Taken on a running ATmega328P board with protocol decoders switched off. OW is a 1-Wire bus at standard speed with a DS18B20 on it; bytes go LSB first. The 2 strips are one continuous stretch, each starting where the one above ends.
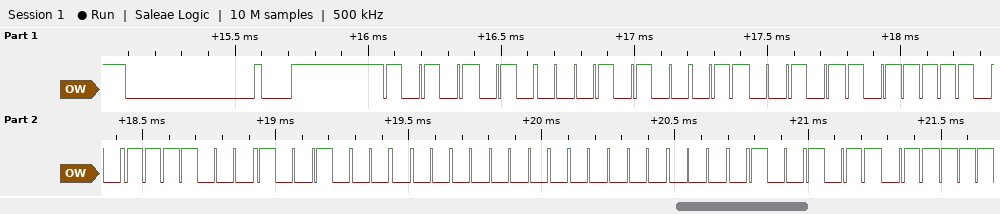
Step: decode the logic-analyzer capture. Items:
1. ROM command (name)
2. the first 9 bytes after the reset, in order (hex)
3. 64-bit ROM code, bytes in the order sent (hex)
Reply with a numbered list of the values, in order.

1. Match ROM
2. 55 28 A6 7D 1E 09 00 00 D2
3. 28 A6 7D 1E 09 00 00 D2
